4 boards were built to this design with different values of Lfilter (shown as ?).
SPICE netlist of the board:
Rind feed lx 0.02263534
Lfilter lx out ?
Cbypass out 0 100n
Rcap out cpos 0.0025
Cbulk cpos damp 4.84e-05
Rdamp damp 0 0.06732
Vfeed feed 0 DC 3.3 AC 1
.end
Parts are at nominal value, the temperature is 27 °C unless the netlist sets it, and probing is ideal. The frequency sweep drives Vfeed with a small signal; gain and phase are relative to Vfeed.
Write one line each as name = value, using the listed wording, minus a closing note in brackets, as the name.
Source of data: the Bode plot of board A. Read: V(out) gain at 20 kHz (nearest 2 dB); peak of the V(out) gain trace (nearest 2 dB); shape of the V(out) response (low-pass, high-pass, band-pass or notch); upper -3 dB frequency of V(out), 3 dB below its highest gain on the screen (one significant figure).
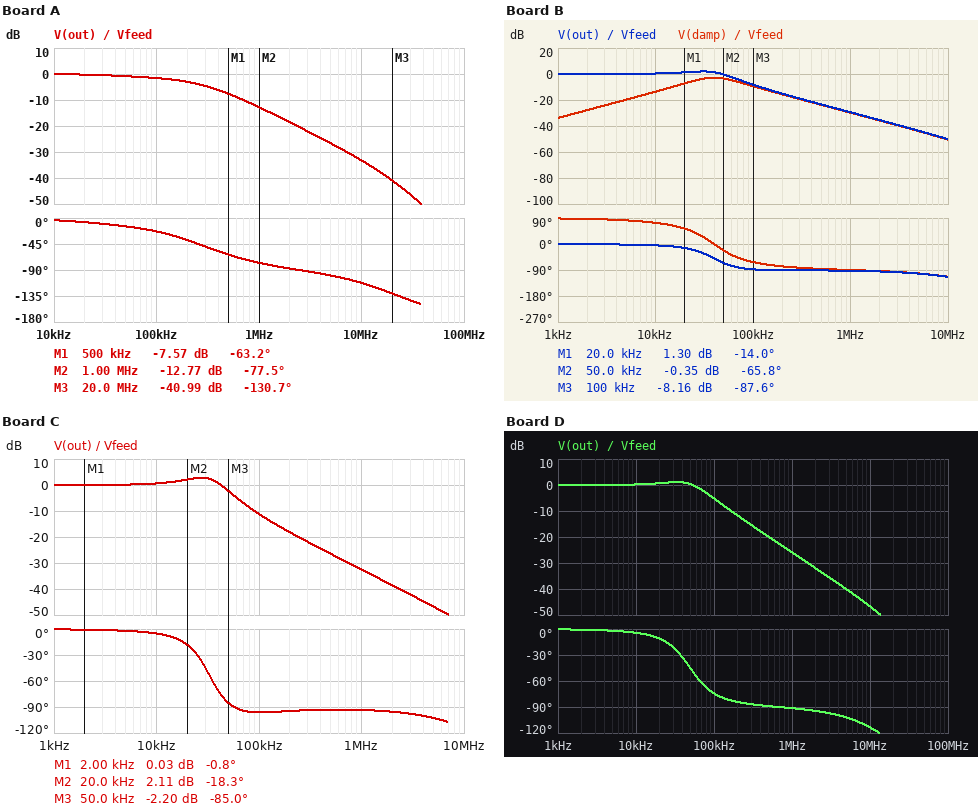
V(out) gain at 20 kHz = 0 dB
peak of the V(out) gain trace = 0 dB
shape of the V(out) response = low-pass
upper -3 dB frequency of V(out), 3 dB below its highest gain on the screen = 200 kHz
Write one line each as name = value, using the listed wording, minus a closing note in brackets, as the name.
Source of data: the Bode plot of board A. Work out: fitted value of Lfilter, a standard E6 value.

fitted value of Lfilter, a standard E6 value = 47 nH
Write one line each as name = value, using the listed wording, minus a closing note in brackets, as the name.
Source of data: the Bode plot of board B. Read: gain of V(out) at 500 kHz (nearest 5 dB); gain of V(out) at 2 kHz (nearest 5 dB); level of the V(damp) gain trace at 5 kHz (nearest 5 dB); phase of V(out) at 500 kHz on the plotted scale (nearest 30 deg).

gain of V(out) at 500 kHz = -25 dB
gain of V(out) at 2 kHz = 0 dB
level of the V(damp) gain trace at 5 kHz = -20 dB
phase of V(out) at 500 kHz on the plotted scale = -90 deg
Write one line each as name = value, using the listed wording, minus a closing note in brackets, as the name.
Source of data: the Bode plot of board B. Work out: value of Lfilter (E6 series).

value of Lfilter = 330 nH
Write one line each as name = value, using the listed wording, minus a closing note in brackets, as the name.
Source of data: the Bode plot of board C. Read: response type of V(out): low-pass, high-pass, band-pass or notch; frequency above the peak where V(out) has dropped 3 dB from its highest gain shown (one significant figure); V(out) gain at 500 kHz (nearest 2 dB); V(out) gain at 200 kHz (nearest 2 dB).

response type of V(out): low-pass, high-pass, band-pass or notch = low-pass
frequency above the peak where V(out) has dropped 3 dB from its highest gain shown = 40 kHz
V(out) gain at 500 kHz = -26 dB
V(out) gain at 200 kHz = -18 dB
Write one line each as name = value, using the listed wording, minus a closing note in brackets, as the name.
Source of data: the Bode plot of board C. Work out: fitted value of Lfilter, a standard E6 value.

fitted value of Lfilter, a standard E6 value = 470 nH
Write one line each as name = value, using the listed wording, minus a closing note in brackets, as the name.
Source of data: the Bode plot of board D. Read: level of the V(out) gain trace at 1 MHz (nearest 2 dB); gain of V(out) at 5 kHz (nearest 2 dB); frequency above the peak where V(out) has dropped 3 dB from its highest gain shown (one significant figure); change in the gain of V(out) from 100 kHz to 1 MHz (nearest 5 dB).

level of the V(out) gain trace at 1 MHz = -26 dB
gain of V(out) at 5 kHz = 0 dB
frequency above the peak where V(out) has dropped 3 dB from its highest gain shown = 70 kHz
change in the gain of V(out) from 100 kHz to 1 MHz = -20 dB
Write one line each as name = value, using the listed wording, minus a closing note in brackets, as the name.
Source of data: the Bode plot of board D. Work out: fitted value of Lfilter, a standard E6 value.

fitted value of Lfilter, a standard E6 value = 220 nH
